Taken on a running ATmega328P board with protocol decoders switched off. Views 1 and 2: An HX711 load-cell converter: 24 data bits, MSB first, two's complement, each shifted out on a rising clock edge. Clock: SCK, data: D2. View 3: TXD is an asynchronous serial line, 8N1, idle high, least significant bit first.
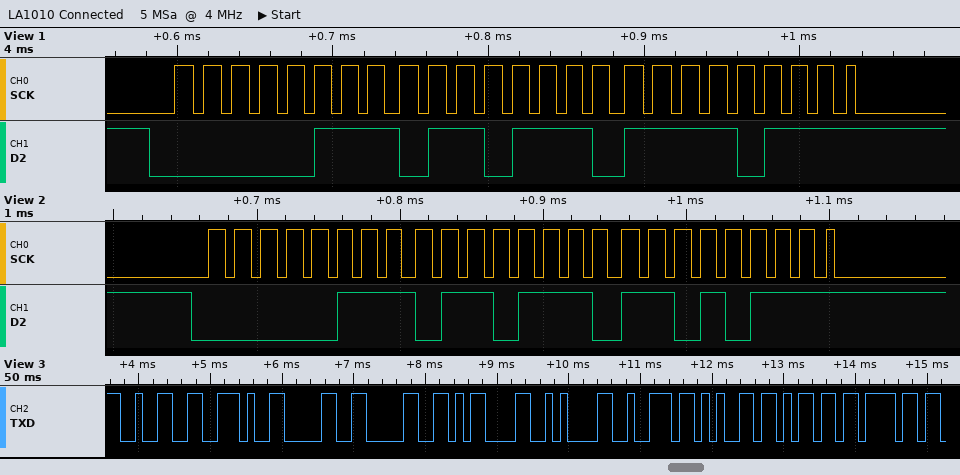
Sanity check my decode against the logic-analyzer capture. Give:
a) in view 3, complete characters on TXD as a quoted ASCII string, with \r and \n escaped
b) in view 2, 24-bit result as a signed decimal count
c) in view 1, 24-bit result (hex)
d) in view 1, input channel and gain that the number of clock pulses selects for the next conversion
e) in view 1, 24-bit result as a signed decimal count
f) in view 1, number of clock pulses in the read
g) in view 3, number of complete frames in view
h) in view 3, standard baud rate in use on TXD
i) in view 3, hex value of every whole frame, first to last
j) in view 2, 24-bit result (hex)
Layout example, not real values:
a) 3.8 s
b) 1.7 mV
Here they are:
a) "2.00\r\nremo"
b) 487127
c) 0x076EF7
d) channel A, gain 128
e) 487159
f) 25
g) 10
h) 9600 baud
i) 32 2E 30 30 0D 0A 72 65 6D 6F
j) 0x076ED7
